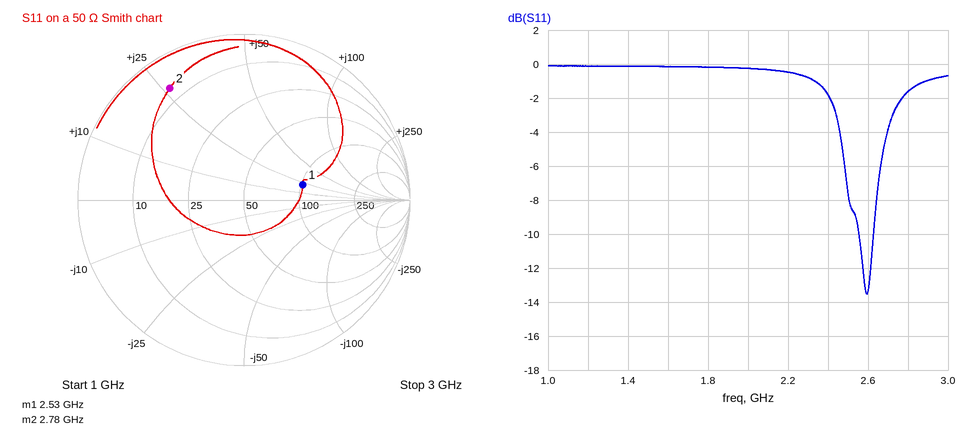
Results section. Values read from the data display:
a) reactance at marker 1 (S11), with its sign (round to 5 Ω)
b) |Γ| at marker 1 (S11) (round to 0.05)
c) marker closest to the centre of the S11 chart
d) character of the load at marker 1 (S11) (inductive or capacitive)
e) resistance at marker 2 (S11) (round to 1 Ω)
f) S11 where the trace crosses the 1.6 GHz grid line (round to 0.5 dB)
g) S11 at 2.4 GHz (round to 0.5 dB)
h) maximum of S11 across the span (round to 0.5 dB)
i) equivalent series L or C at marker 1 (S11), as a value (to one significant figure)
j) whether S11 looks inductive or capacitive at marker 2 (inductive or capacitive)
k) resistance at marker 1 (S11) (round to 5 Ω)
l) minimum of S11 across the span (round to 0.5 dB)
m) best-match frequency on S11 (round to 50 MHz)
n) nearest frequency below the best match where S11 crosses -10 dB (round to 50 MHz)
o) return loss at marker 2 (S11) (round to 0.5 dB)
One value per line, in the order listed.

+20 Ω
0.35
marker 1
inductive
7 Ω
0.0 dB
-2.0 dB
0.0 dB
1 nH
inductive
100 Ω
-13.5 dB
2.60 GHz
2.55 GHz
2.0 dB
